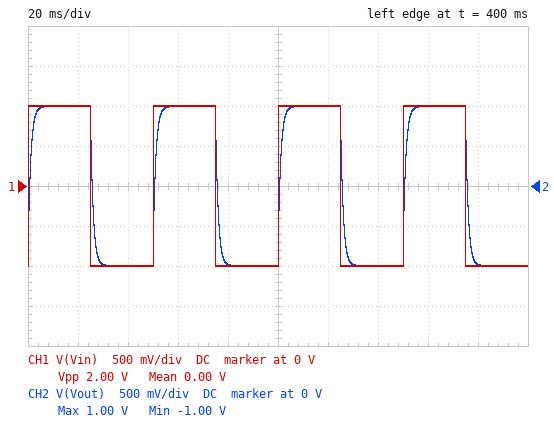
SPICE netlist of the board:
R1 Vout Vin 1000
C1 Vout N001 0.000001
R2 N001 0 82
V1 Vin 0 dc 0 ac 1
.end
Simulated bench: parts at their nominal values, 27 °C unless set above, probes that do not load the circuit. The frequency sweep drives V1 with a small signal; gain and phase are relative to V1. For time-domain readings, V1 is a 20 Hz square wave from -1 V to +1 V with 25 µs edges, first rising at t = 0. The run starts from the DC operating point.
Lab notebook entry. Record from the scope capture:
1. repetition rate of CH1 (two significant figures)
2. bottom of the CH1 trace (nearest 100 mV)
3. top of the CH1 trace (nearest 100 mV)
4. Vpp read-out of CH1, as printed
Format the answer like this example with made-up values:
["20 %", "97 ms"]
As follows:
["20 Hz", "-1.0 V", "1.0 V", "2.00 V"]
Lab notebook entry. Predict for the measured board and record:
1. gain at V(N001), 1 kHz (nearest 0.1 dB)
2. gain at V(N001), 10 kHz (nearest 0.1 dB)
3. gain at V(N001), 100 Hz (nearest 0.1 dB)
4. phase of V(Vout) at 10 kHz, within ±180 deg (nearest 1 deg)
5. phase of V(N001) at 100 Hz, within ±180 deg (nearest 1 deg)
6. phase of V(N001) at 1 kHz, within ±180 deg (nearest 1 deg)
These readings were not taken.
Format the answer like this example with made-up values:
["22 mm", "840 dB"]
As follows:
["-22.5 dB", "-22.4 dB", "-27.4 dB", "-10 deg", "56 deg", "8 deg"]
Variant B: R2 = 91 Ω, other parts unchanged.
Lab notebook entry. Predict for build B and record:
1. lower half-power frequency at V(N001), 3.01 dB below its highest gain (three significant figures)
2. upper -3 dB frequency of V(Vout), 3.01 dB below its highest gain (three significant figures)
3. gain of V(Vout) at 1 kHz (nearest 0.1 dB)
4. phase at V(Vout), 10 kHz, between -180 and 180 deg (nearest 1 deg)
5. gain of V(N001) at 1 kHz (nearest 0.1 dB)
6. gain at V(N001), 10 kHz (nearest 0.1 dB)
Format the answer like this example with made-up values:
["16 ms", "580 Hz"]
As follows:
["146 Hz", "147 Hz", "-15.6 dB", "-9 deg", "-21.7 dB", "-21.6 dB"]
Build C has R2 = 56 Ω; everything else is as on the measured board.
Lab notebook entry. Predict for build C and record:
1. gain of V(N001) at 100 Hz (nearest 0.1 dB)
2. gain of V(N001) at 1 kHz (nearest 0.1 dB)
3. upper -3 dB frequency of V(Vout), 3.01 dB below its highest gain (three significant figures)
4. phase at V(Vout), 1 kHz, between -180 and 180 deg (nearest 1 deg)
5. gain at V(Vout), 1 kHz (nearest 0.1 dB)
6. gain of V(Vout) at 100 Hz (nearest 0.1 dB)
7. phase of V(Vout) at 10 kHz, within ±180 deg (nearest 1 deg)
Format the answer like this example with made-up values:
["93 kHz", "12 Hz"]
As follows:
["-30.7 dB", "-25.6 dB", "151 Hz", "-62 deg", "-16.0 dB", "-1.6 dB", "-15 deg"]
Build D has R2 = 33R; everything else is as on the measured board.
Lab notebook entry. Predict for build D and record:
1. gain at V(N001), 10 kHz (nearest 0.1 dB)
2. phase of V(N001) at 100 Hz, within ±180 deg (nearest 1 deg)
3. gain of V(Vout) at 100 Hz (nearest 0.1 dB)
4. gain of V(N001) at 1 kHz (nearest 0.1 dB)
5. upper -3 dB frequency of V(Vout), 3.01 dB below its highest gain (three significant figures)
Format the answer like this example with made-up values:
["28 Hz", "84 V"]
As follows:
["-29.9 dB", "57 deg", "-1.5 dB", "-30.0 dB", "154 Hz"]
